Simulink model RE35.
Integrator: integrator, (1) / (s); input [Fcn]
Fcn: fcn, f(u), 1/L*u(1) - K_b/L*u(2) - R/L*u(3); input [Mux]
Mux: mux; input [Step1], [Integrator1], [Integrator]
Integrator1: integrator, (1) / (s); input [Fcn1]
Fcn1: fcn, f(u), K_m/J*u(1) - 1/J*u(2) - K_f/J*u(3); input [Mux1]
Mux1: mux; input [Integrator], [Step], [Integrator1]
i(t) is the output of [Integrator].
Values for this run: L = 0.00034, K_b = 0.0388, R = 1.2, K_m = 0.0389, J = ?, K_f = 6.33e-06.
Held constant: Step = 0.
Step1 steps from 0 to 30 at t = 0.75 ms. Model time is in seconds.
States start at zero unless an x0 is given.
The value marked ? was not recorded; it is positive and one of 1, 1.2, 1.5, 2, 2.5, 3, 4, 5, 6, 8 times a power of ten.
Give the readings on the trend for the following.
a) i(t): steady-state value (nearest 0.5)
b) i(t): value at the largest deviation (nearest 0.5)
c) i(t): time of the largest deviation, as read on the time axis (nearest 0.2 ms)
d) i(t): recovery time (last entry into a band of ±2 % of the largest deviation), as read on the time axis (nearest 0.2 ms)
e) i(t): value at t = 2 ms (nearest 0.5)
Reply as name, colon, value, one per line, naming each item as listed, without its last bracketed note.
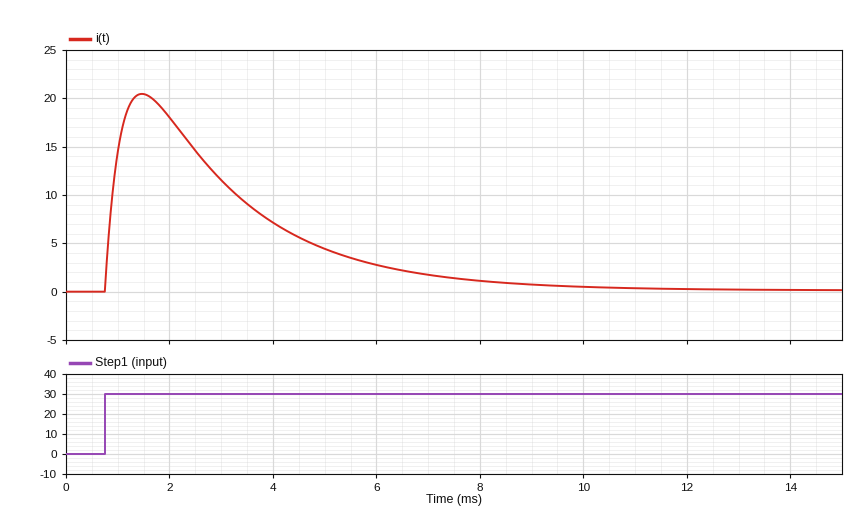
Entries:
i(t): steady-state value: 0.0
i(t): value at the largest deviation: 20.5
i(t): time of the largest deviation, as read on the time axis: 1.4 ms
i(t): recovery time (last entry into a band of ±2 % of the largest deviation), as read on the time axis: 9.8 ms
i(t): value at t = 2 ms: 18.0
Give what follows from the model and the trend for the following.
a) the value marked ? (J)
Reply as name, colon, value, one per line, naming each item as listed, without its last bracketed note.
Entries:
the value marked ?: 3e-06
